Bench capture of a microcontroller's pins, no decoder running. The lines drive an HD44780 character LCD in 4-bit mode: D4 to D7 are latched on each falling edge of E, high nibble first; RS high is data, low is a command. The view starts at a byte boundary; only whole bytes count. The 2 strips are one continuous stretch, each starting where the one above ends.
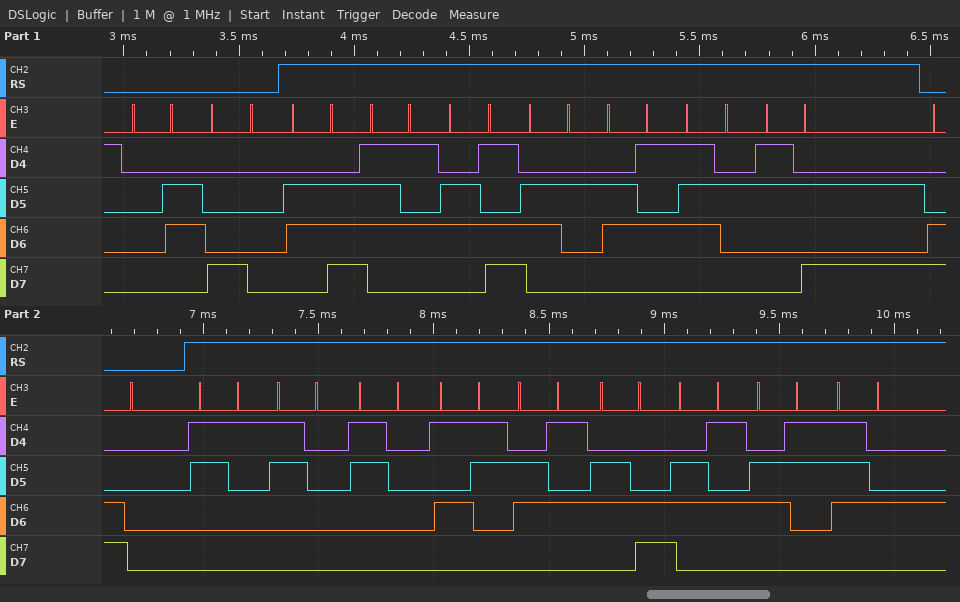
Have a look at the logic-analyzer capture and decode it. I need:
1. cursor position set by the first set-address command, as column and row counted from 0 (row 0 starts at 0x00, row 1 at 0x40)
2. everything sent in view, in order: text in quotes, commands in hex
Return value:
column 0, row 0
0x06 0x80 "number:" 0xC0 "100Select"
